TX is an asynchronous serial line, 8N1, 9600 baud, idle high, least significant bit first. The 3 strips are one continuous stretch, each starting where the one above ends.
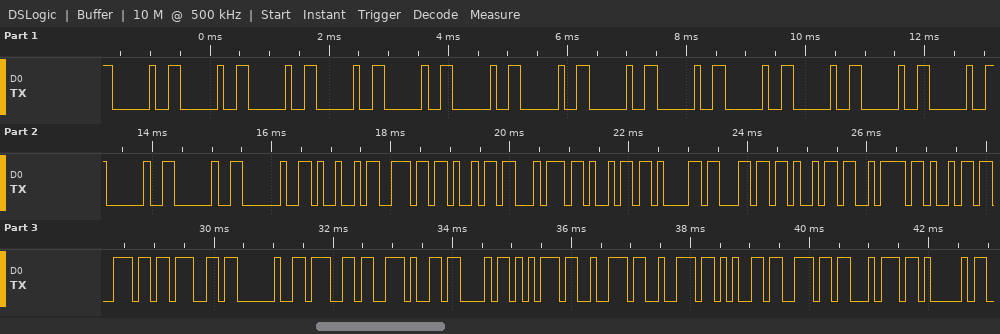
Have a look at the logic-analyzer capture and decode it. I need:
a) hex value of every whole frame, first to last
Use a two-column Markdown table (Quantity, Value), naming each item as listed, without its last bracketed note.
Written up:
| Quantity | Value |
|---|---|
| hex value of every whole frame, first to last | 20 20 20 20 20 20 20 20 20 20 20 20 20 20 20 20 49 6E 69 74 69 61 6C 69 7A 69 6E 67 20 67 2E 43 75 72 72 65 6E 74 41 |
